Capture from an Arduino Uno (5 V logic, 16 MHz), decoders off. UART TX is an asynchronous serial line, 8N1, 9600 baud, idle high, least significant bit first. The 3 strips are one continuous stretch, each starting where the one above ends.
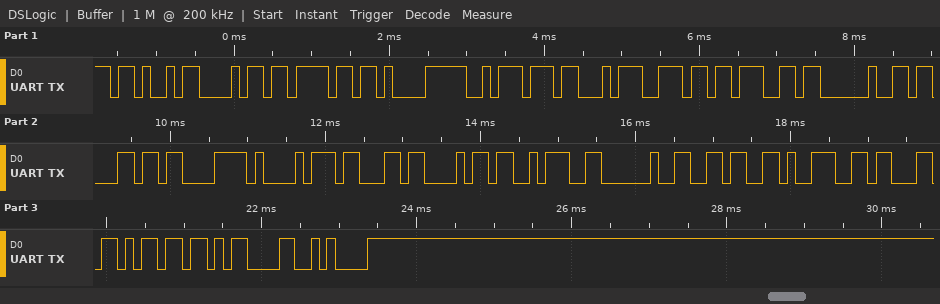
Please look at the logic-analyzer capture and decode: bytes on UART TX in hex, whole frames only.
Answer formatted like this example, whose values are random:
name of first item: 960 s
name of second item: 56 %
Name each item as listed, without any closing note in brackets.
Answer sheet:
bytes on UART TX in hex, whole frames only: 4B 68 6F E1 BA A3 6E 67 20 63 C3 A1 63 68 3A 20 36 39 63 6D 0D 0A
